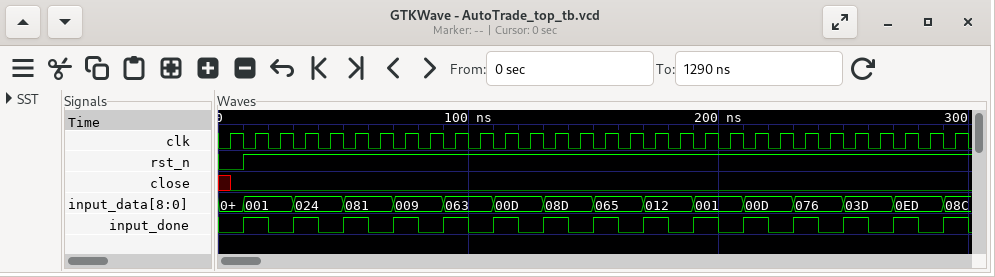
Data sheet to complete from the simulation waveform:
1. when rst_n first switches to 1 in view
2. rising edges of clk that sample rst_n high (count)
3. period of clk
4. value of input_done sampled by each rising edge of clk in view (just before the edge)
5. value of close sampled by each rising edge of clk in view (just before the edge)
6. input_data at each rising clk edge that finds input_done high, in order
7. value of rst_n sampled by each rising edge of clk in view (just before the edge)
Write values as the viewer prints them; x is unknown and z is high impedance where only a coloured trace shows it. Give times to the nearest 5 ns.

10 ns
29
10 ns
0 1 0 1 0 1 0 1 0 1 0 1 0 1 0 1 0 1 0 1 0 1 0 1 0 1 0 1 0 1
x 0 0 0 0 0 0 0 0 0 0 0 0 0 0 0 0 0 0 0 0 0 0 0 0 0 0 0 0 0
001, 024, 081, 009, 063, 00D, 08D, 065, 012, 001, 00D, 076, 03D, 0ED, 08C
0 1 1 1 1 1 1 1 1 1 1 1 1 1 1 1 1 1 1 1 1 1 1 1 1 1 1 1 1 1
